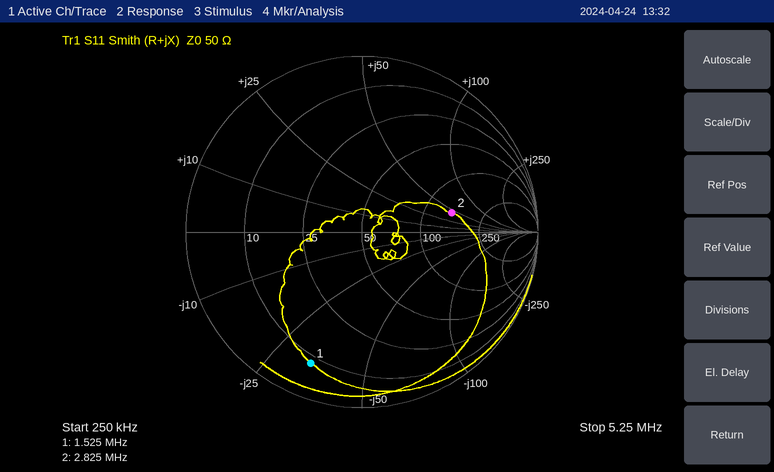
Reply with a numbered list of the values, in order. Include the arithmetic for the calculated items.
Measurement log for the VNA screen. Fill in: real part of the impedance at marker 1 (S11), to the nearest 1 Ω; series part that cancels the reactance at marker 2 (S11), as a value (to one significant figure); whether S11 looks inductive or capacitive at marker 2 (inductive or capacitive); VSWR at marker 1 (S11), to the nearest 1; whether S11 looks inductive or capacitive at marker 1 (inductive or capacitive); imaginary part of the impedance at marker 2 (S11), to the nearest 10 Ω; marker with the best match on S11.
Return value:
1. 8 Ω
2. C = 1/(2π × 2.825 MHz × 40 Ω) ≈ 1 nF
3. inductive
4. 9
5. capacitive
6. +40 Ω
7. marker 2
